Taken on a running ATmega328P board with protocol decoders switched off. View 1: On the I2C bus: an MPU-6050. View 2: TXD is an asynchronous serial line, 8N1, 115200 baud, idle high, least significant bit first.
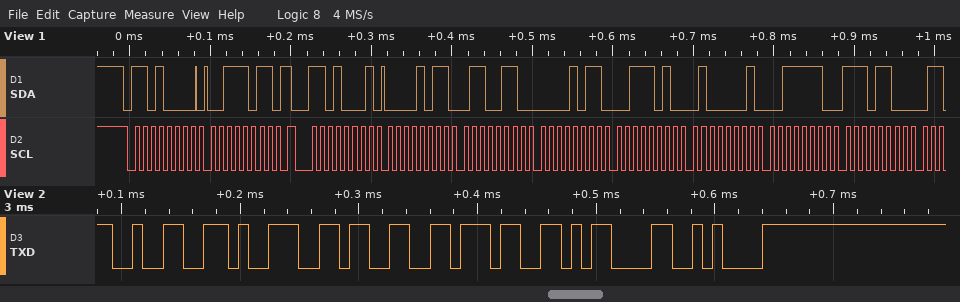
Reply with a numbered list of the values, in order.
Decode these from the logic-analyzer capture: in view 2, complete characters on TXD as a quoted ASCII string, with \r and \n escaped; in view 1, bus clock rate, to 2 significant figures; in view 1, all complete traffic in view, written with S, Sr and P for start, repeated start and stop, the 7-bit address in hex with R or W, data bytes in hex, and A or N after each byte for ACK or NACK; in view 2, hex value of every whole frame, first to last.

1. "2937\r\n"
2. 100 kHz
3. S 68W A 3B A Sr 68R A 0B A 66 A 0B A 3A A 41 A 3E A EC A
4. 0x32 0x39 0x33 0x37 0x0D 0x0A
